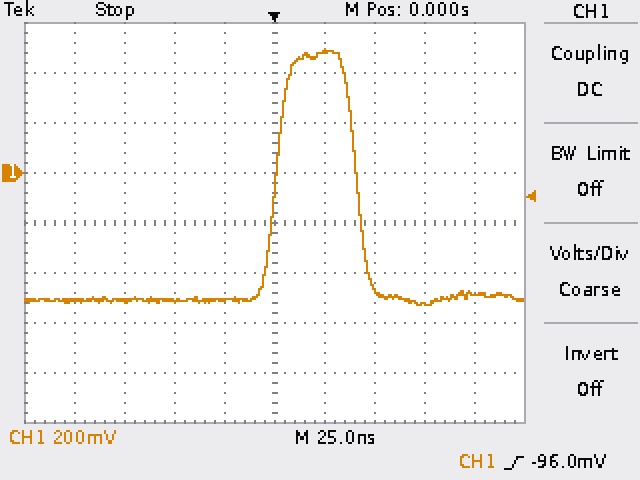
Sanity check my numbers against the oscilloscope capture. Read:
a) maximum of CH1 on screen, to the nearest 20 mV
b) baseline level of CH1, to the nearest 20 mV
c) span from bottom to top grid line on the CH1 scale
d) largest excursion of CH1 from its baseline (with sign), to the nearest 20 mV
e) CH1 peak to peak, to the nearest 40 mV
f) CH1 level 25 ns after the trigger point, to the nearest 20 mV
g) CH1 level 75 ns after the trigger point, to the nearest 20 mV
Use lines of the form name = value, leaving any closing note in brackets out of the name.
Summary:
maximum of CH1 on screen, to the nearest 20 mV = 500 mV
baseline level of CH1, to the nearest 20 mV = -500 mV
span from bottom to top grid line on the CH1 scale = 1.6 V
largest excursion of CH1 from its baseline (with sign), to the nearest 20 mV = +1.00 V
CH1 peak to peak, to the nearest 40 mV = 1.04 V
CH1 level 25 ns after the trigger point, to the nearest 20 mV = 480 mV
CH1 level 75 ns after the trigger point, to the nearest 20 mV = -520 mV
